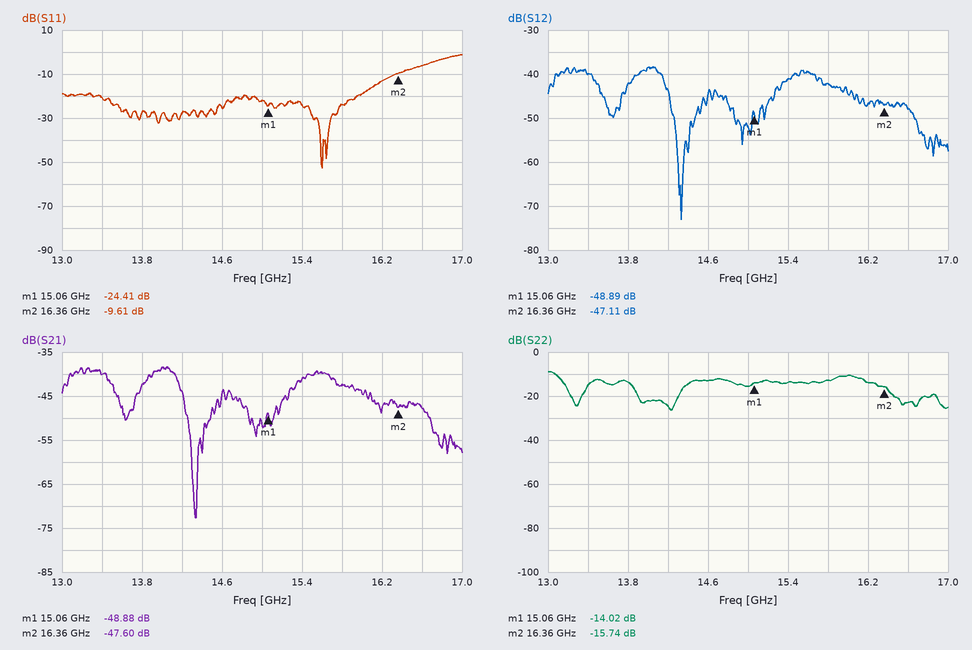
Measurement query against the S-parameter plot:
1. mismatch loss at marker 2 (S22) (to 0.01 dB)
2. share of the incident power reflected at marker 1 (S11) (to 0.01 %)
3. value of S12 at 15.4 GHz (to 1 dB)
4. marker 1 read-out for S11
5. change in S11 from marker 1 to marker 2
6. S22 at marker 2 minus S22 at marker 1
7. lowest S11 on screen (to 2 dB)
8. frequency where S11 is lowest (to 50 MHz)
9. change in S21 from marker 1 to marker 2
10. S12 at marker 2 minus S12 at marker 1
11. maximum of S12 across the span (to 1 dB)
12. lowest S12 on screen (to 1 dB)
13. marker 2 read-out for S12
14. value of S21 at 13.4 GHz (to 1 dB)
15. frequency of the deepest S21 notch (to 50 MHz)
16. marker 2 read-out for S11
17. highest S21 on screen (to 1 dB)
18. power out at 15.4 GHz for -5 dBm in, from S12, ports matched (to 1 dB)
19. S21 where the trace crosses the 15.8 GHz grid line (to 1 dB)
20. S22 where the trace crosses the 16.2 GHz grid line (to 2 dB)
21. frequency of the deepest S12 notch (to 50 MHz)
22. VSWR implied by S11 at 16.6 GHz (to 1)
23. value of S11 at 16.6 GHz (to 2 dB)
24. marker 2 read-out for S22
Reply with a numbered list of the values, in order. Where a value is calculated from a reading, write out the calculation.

1. −10 log10(1 − 10^(-15.74/10)) ≈ 0.12 dB
2. 10^(-24.41/10) ≈ 0.36 %
3. -41 dB
4. -24.41 dB
5. -9.61 − (-24.41) = 14.80 dB
6. -15.74 − (-14.02) = -1.72 dB
7. -52 dB
8. 15.60 GHz
9. -47.6 − (-48.88) = 1.28 dB
10. -47.11 − (-48.89) = 1.78 dB
11. -38 dB
12. -73 dB
13. -47.11 dB
14. -40 dB
15. 14.35 GHz
16. -9.61 dB
17. -38 dB
18. -5 dBm + (-41 dB) = -46 dBm
19. -42 dB
20. -14 dB
21. 14.35 GHz
22. |Γ| = 10^(-6/20) = 0.5012; VSWR = (1 + 0.5012)/(1 − 0.5012) ≈ 3
23. -6 dB
24. -15.74 dB
